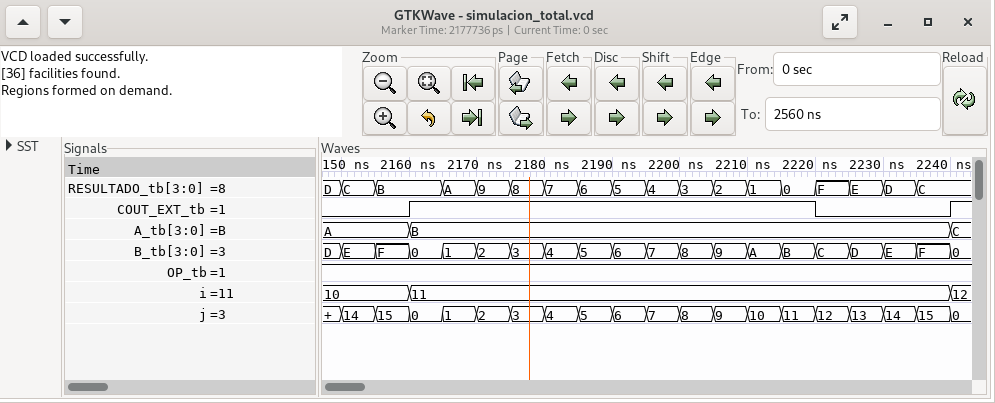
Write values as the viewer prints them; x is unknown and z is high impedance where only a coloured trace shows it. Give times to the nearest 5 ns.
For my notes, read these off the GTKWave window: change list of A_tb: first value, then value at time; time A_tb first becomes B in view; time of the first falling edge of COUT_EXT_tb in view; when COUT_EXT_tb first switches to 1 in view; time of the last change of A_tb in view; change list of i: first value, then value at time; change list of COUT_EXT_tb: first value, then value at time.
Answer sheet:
A, B at 2160 ns, C at 2240 ns
2160 ns
2220 ns
2160 ns
2240 ns
10, 11 at 2160 ns, 12 at 2240 ns
0, 1 at 2160 ns, 0 at 2220 ns, 1 at 2240 ns
